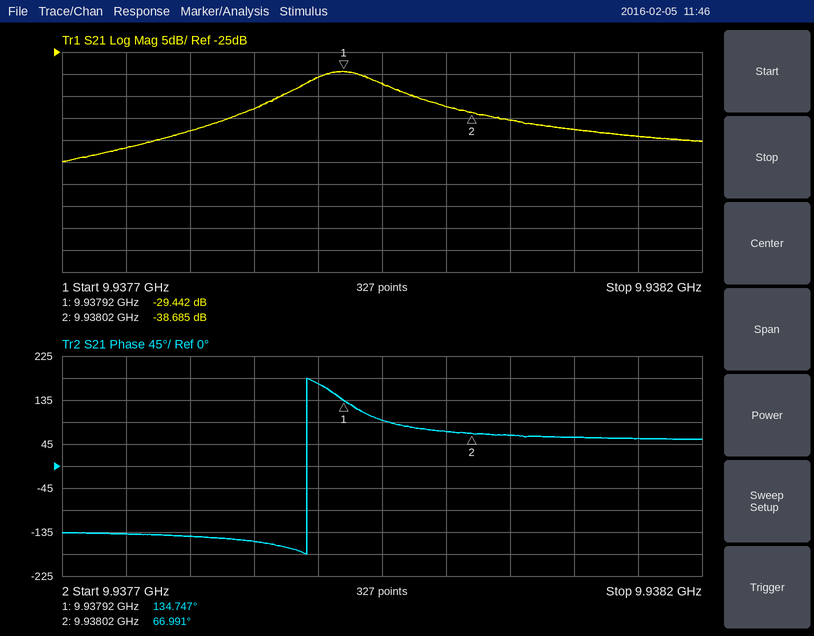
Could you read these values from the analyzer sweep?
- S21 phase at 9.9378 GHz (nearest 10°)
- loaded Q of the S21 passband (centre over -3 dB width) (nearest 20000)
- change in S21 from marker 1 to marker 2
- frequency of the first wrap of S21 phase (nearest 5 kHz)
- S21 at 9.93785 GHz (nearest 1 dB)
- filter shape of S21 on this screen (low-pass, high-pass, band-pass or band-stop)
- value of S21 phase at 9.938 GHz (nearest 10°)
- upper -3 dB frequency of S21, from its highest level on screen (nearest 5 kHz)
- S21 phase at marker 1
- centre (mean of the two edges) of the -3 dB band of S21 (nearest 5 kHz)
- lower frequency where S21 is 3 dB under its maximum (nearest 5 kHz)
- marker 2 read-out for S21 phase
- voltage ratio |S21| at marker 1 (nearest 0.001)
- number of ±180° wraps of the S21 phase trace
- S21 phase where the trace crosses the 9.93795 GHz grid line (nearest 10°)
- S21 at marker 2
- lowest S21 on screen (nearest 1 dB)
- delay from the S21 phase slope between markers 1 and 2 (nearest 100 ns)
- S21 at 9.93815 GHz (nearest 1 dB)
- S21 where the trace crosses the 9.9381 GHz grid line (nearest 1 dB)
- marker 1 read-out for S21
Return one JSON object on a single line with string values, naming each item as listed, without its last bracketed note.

{"S21 phase at 9.9378 GHz": "-140°", "loaded Q of the S21 passband (centre over -3 dB width)": "160000", "change in S21 from marker 1 to marker 2": "-9.243 dB", "frequency of the first wrap of S21 phase": "9.937890 GHz", "S21 at 9.93785 GHz": "-38 dB", "filter shape of S21 on this screen": "band-pass", "value of S21 phase at 9.938 GHz": "70°", "upper -3 dB frequency of S21, from its highest level on screen": "9.937950 GHz", "S21 phase at marker 1": "134.747°", "centre (mean of the two edges) of the -3 dB band of S21": "9.937920 GHz", "lower frequency where S21 is 3 dB under its maximum": "9.937890 GHz", "marker 2 read-out for S21 phase": "66.991°", "voltage ratio |S21| at marker 1": "0.034", "number of ±180° wraps of the S21 phase trace": "1", "S21 phase where the trace crosses the 9.93795 GHz grid line": "90°", "S21 at marker 2": "-38.685 dB", "lowest S21 on screen": "-50 dB", "delay from the S21 phase slope between markers 1 and 2": "1.9 µs", "S21 at 9.93815 GHz": "-44 dB", "S21 where the trace crosses the 9.9381 GHz grid line": "-43 dB", "marker 1 read-out for S21": "-29.442 dB"}
